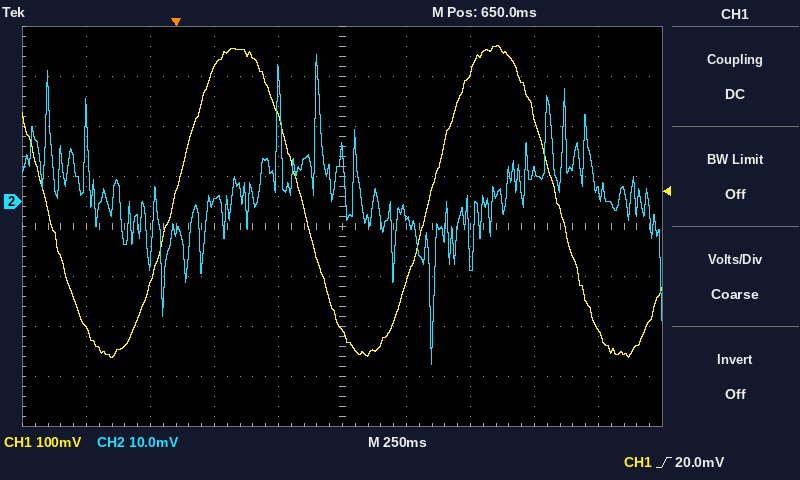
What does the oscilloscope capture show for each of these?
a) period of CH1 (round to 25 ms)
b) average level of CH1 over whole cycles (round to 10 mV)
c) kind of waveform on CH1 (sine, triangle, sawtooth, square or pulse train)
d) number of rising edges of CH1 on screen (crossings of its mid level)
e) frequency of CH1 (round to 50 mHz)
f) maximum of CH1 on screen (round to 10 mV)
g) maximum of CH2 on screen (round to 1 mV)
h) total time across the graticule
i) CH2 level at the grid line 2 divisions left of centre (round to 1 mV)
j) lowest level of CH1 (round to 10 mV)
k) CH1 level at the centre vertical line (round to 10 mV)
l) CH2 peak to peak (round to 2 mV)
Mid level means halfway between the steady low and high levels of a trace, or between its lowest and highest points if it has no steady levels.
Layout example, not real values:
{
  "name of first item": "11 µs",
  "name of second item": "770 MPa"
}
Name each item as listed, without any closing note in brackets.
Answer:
{
  "period of CH1": "1.000 s",
  "average level of CH1 over whole cycles": "0 mV",
  "kind of waveform on CH1": "sine",
  "number of rising edges of CH1 on screen": "2",
  "frequency of CH1": "1.00 Hz",
  "maximum of CH1 on screen": "310 mV",
  "maximum of CH2 on screen": "29 mV",
  "total time across the graticule": "2.5 s",
  "CH2 level at the grid line 2 divisions left of centre": "0 mV",
  "lowest level of CH1": "-310 mV",
  "CH1 level at the centre vertical line": "-260 mV",
  "CH2 peak to peak": "62 mV"
}
